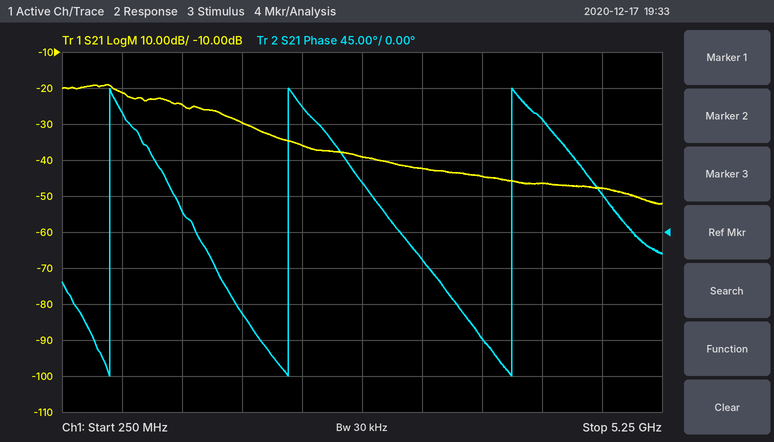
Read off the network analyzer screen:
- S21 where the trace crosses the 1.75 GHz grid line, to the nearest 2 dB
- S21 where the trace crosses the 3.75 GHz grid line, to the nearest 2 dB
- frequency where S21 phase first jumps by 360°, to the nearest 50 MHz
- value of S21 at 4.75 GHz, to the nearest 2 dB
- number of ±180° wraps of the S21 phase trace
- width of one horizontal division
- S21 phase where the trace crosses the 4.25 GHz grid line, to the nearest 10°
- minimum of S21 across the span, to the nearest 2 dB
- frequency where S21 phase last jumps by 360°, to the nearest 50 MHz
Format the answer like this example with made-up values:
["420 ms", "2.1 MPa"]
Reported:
["-30 dB", "-44 dB", "650 MHz", "-48 dB", "3", "500 MHz", "140°", "-52 dB", "4.00 GHz"]
